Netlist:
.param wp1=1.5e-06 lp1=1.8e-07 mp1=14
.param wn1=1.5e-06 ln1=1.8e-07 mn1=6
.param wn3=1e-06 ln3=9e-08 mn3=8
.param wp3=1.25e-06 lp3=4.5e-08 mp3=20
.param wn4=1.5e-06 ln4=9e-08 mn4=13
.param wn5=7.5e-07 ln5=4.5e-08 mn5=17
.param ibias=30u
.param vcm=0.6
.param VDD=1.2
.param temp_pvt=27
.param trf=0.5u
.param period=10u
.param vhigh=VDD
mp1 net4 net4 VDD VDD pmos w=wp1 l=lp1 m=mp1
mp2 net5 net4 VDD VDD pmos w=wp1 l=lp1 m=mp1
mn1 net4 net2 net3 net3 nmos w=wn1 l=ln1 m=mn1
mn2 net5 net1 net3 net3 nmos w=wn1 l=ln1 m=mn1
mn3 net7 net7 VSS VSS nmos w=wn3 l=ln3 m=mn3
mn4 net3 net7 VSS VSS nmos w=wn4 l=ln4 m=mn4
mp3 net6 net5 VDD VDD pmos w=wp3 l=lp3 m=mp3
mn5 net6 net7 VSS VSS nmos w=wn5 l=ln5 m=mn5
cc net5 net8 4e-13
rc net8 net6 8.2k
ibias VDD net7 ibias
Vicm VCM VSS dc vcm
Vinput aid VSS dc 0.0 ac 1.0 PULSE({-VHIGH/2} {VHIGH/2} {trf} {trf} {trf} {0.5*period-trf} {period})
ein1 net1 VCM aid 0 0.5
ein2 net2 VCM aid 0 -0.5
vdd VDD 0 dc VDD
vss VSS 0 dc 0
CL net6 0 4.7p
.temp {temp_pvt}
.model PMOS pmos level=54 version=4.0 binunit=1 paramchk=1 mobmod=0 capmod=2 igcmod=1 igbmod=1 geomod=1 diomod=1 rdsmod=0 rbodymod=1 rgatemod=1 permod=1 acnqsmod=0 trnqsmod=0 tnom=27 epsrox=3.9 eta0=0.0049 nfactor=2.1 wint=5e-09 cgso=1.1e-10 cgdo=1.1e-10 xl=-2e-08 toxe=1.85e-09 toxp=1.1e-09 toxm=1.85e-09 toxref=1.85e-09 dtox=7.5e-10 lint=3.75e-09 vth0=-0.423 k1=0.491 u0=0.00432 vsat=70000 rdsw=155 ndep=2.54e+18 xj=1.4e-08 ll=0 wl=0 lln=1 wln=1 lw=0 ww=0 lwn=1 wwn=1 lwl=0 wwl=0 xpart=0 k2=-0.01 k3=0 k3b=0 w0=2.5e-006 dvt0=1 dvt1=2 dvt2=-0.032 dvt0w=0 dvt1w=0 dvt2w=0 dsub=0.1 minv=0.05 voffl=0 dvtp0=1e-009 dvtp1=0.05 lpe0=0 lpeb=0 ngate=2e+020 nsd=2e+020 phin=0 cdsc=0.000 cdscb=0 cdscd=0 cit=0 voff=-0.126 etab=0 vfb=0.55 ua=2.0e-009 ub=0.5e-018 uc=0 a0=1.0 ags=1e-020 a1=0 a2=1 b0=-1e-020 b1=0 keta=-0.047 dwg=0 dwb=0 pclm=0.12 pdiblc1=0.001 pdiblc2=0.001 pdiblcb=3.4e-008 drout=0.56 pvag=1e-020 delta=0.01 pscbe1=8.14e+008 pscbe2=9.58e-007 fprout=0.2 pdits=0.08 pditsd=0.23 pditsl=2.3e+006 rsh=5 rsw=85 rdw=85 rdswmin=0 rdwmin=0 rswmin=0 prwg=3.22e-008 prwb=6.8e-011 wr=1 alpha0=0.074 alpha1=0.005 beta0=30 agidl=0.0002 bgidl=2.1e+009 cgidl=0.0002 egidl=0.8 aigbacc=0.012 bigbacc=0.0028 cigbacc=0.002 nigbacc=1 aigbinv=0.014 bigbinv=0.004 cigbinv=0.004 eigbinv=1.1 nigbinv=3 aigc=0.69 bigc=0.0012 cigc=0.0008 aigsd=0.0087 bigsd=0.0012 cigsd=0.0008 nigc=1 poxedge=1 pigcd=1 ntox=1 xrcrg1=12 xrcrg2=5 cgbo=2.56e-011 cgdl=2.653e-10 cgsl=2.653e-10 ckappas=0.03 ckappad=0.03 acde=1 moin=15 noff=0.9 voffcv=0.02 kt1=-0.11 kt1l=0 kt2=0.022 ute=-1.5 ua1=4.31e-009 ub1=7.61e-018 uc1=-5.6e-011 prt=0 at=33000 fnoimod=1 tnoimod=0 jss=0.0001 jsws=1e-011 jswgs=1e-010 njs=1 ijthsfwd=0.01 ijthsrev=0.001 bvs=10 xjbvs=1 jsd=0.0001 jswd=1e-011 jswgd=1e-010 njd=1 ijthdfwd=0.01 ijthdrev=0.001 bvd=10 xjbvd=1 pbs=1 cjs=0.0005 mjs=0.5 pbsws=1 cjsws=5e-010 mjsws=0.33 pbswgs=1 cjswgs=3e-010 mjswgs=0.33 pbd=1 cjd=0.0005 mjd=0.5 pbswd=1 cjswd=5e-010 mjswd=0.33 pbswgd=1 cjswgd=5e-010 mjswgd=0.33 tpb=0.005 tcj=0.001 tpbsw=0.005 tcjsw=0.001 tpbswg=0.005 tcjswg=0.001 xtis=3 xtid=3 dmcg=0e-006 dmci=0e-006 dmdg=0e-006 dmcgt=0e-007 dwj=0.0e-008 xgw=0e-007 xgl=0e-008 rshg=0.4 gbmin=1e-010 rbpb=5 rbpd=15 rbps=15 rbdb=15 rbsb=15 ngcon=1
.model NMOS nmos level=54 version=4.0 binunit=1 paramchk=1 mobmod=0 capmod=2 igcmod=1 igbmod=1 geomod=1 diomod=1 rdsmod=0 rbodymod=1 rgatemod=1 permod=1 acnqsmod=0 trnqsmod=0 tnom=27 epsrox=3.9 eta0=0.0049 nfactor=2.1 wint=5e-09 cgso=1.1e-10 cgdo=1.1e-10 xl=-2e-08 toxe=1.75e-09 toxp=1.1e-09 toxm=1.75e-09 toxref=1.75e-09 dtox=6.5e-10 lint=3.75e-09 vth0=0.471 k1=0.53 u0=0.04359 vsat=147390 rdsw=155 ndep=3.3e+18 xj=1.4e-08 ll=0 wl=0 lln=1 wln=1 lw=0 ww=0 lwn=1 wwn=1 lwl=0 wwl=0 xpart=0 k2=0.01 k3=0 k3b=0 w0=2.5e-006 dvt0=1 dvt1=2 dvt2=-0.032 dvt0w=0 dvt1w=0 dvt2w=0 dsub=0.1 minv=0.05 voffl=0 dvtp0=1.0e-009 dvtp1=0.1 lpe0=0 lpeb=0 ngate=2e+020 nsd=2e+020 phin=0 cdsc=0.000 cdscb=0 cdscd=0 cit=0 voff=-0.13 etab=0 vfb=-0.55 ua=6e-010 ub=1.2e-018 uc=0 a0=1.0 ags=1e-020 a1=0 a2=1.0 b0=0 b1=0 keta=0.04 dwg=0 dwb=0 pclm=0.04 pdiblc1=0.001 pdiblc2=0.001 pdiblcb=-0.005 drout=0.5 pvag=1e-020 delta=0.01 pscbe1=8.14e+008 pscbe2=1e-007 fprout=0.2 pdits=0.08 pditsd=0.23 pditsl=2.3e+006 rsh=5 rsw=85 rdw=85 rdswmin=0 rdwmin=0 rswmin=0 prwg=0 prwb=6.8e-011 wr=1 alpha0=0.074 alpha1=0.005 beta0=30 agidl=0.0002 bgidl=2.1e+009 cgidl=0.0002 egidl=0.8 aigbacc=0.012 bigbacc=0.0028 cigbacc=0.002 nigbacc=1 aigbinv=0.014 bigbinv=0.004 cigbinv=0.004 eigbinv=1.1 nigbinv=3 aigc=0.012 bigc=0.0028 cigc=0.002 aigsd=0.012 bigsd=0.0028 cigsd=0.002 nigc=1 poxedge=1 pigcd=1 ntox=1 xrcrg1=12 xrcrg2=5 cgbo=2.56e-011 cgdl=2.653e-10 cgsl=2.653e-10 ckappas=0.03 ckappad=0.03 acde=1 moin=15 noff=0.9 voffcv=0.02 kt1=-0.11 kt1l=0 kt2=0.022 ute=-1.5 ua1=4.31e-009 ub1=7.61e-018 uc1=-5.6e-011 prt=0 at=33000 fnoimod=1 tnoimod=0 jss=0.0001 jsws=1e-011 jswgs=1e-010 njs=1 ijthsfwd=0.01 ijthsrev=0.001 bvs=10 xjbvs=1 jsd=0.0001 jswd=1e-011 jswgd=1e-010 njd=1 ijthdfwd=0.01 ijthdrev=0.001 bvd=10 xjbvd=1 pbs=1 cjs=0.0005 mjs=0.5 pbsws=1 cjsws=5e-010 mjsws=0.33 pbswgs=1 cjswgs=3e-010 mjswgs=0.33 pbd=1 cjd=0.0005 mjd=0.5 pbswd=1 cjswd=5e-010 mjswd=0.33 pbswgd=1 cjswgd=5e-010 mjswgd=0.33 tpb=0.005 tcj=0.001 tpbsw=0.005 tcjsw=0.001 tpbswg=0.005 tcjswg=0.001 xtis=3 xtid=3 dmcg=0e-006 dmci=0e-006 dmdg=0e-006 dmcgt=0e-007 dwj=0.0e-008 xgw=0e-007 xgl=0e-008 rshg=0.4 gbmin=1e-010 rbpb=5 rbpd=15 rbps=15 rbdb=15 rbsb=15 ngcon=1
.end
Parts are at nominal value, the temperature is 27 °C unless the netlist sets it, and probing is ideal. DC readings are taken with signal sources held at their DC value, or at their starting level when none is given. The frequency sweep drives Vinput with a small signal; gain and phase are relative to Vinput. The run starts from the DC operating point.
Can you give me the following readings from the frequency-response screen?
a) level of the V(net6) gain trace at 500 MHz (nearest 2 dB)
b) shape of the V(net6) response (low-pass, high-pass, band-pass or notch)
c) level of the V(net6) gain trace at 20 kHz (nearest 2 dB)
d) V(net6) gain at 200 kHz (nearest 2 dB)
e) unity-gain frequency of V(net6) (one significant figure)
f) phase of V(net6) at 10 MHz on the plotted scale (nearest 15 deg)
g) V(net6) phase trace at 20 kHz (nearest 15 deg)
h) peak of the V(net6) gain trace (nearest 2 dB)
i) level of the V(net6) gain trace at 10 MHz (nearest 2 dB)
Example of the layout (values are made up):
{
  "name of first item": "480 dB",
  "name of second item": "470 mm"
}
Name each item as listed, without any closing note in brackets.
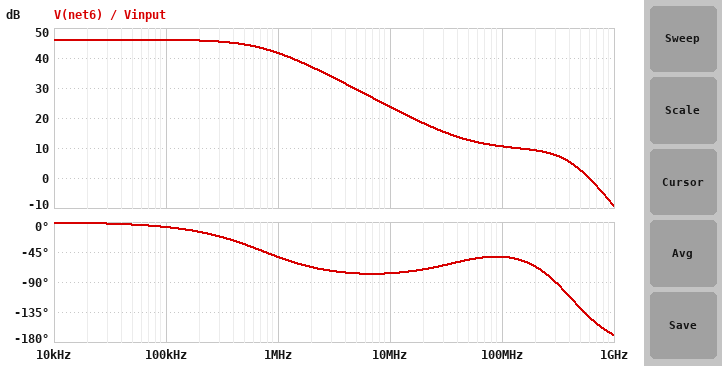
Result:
{
  "level of the V(net6) gain trace at 500 MHz": "2 dB",
  "shape of the V(net6) response": "low-pass",
  "level of the V(net6) gain trace at 20 kHz": "46 dB",
  "V(net6) gain at 200 kHz": "46 dB",
  "unity-gain frequency of V(net6)": "600 MHz",
  "phase of V(net6) at 10 MHz on the plotted scale": "-75 deg",
  "V(net6) phase trace at 20 kHz": "0 deg",
  "peak of the V(net6) gain trace": "46 dB",
  "level of the V(net6) gain trace at 10 MHz": "24 dB"
}
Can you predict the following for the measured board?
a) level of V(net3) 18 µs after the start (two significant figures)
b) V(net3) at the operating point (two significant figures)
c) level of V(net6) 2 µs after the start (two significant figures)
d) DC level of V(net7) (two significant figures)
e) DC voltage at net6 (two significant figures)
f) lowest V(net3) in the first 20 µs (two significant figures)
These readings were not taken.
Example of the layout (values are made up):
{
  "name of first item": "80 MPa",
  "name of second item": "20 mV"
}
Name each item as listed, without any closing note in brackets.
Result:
{
  "level of V(net3) 18 µs after the start": "410 mV",
  "V(net3) at the operating point": "150 mV",
  "level of V(net6) 2 µs after the start": "1.1 V",
  "DC level of V(net7)": "400 mV",
  "DC voltage at net6": "750 mV",
  "lowest V(net3) in the first 20 µs": "2.0 mV"
}
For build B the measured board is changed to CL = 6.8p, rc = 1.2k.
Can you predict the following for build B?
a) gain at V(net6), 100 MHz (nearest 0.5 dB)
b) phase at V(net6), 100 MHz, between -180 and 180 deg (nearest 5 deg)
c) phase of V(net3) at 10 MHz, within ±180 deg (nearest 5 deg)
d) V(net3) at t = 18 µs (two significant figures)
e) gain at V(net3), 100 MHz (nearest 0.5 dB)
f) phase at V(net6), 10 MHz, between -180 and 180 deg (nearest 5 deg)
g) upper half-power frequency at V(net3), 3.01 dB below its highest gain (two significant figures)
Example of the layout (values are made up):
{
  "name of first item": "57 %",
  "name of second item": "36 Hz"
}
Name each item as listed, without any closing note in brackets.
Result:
{
  "gain at V(net6), 100 MHz": "3.5 dB",
  "phase at V(net6), 100 MHz, between -180 and 180 deg": "-100 deg",
  "phase of V(net3) at 10 MHz, within ±180 deg": "115 deg",
  "V(net3) at t = 18 µs": "410 mV",
  "gain at V(net3), 100 MHz": "-42.5 dB",
  "phase at V(net6), 10 MHz, between -180 and 180 deg": "-85 deg",
  "upper half-power frequency at V(net3), 3.01 dB below its highest gain": "760 kHz"
}
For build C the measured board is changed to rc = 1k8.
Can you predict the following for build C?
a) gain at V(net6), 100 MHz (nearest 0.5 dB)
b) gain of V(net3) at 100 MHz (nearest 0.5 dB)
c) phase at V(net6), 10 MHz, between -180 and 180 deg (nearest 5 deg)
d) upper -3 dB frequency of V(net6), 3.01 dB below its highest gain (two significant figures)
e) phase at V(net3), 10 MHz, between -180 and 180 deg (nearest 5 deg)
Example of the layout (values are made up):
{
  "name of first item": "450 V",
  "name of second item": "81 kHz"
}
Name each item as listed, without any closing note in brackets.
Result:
{
  "gain at V(net6), 100 MHz": "4.0 dB",
  "gain of V(net3) at 100 MHz": "-42.5 dB",
  "phase at V(net6), 10 MHz, between -180 and 180 deg": "-85 deg",
  "upper -3 dB frequency of V(net6), 3.01 dB below its highest gain": "760 kHz",
  "phase at V(net3), 10 MHz, between -180 and 180 deg": "115 deg"
}
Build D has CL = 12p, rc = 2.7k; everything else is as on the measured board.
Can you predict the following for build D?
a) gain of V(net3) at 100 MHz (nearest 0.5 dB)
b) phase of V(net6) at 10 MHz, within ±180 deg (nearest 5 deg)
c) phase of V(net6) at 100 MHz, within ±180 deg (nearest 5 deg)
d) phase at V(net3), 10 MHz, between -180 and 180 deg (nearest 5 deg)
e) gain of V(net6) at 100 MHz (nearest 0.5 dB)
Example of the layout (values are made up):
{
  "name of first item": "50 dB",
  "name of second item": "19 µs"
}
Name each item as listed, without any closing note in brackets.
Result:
{
  "gain of V(net3) at 100 MHz": "-41.0 dB",
  "phase of V(net6) at 10 MHz, within ±180 deg": "-85 deg",
  "phase of V(net6) at 100 MHz, within ±180 deg": "-95 deg",
  "phase at V(net3), 10 MHz, between -180 and 180 deg": "120 deg",
  "gain of V(net6) at 100 MHz": "4.0 dB"
}
